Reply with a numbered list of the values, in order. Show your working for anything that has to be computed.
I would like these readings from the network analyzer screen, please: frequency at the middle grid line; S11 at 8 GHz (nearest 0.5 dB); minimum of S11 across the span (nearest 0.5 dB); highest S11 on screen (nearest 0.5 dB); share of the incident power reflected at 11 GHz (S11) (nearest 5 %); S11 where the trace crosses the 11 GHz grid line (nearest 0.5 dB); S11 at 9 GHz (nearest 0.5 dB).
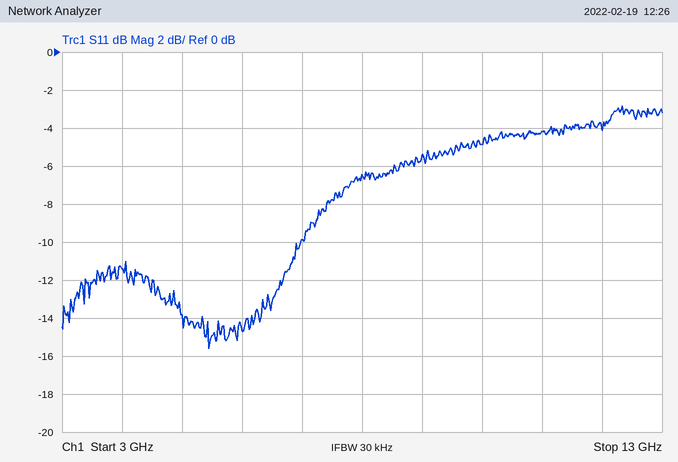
1. 8 GHz
2. -6.5 dB
3. -15.5 dB
4. -3.0 dB
5. 10^(-4/10) ≈ 40 %
6. -4.0 dB
7. -5.5 dB
